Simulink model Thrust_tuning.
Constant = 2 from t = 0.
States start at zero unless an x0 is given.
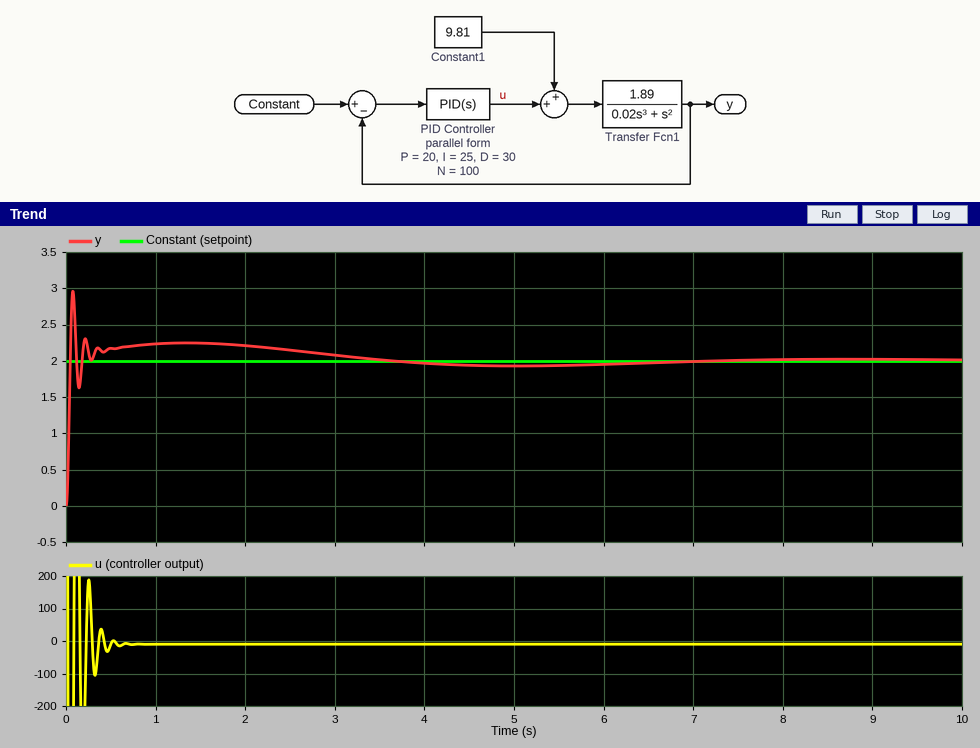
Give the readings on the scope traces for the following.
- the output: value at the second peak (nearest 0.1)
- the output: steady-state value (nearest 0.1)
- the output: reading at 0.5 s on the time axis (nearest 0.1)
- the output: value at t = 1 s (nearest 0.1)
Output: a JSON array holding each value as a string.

["2.3", "2.0", "2.2", "2.2"]
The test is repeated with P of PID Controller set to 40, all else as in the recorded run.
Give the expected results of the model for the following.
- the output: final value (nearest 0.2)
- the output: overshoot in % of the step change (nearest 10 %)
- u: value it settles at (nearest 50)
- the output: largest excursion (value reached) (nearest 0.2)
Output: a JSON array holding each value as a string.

["2.0", "50 %", "0", "3.0"]
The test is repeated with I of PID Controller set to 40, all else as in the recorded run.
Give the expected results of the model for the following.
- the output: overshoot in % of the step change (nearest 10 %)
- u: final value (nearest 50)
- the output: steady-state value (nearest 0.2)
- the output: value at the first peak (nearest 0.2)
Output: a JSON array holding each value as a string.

["50 %", "0", "2.0", "3.0"]
